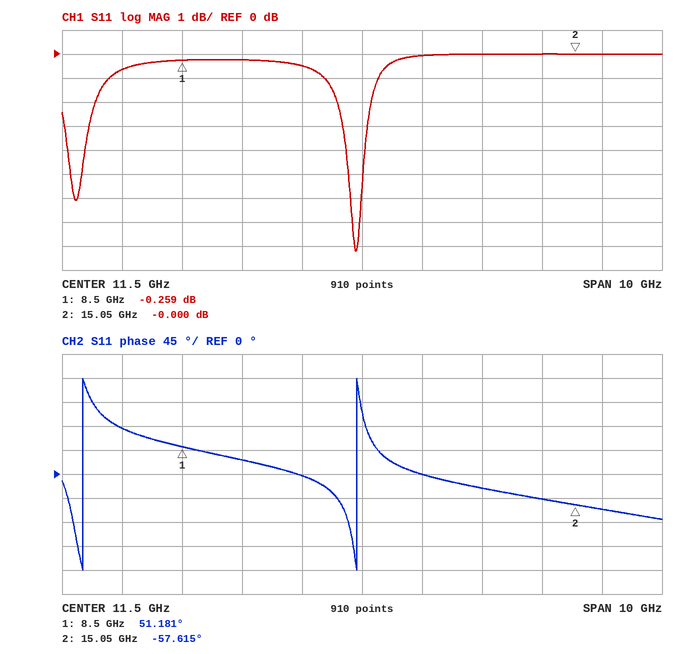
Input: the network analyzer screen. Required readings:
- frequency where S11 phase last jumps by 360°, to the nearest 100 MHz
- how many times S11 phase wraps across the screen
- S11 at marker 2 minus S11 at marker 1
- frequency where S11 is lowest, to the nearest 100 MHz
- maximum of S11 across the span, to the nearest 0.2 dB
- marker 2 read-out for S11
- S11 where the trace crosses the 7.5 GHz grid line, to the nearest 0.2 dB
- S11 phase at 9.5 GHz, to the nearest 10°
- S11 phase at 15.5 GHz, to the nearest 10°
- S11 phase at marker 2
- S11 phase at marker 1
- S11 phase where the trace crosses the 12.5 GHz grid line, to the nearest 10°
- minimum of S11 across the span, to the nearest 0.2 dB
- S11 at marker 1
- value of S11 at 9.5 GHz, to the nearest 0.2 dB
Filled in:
11.4 GHz
2
0.259 dB
11.4 GHz
0.0 dB
-0.000 dB
-0.6 dB
30°
-70°
-57.615°
51.181°
0°
-8.2 dB
-0.259 dB
-0.2 dB
